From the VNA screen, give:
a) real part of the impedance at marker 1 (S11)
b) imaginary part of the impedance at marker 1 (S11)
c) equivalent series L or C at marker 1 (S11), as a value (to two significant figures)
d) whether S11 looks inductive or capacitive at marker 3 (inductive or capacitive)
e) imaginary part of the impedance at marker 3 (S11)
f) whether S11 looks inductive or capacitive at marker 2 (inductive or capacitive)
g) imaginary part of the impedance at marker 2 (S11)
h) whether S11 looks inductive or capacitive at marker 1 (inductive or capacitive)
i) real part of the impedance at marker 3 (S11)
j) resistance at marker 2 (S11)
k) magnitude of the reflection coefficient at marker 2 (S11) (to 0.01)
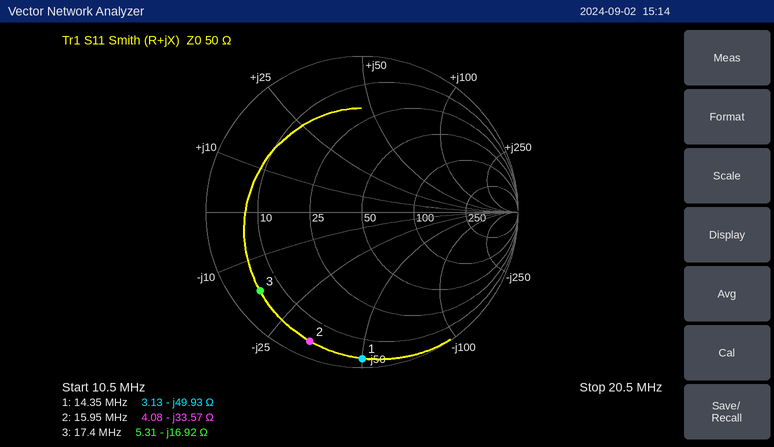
3.13 Ω
-49.93 Ω
220 pF
capacitive
-16.92 Ω
capacitive
-33.57 Ω
capacitive
5.31 Ω
4.08 Ω
0.89
